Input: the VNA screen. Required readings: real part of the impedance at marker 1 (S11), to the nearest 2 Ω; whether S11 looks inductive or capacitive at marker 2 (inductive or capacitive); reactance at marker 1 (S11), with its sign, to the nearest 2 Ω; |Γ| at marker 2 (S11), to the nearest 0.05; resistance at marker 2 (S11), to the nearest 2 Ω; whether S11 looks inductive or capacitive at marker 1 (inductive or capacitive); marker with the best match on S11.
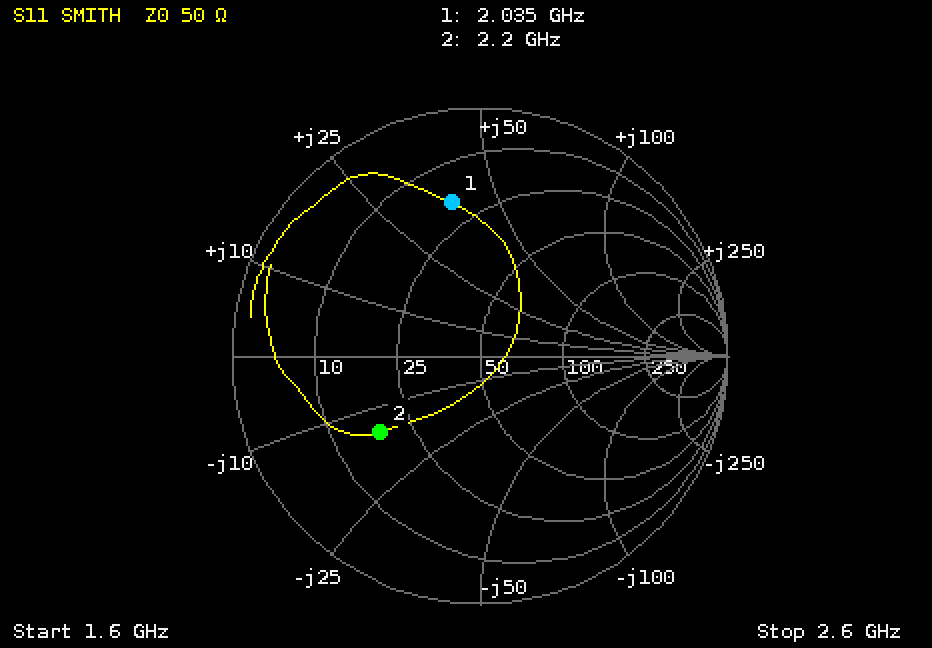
18 Ω
capacitive
+38 Ω
0.50
18 Ω
inductive
marker 2
